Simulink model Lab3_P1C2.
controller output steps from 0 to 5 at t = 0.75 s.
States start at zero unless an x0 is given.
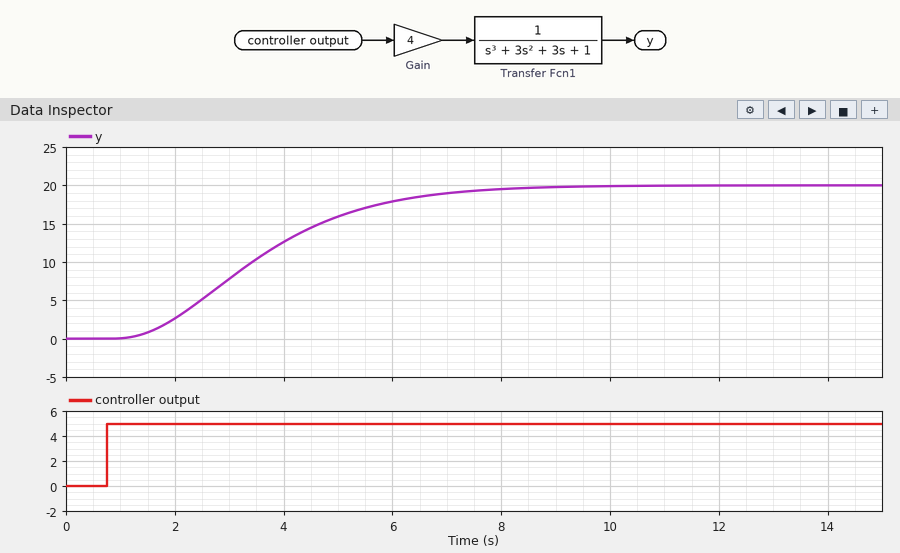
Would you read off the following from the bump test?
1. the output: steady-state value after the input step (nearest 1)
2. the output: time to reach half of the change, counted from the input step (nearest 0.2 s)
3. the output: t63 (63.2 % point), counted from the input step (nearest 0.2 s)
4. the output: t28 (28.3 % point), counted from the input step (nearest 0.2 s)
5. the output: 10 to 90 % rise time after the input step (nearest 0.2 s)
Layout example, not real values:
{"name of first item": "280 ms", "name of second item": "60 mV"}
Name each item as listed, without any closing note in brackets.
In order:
{"the output: steady-state value after the input step": "20", "the output: time to reach half of the change, counted from the input step": "2.6 s", "the output: t63 (63.2 % point), counted from the input step": "3.2 s", "the output: t28 (28.3 % point), counted from the input step": "1.8 s", "the output: 10 to 90 % rise time after the input step": "4.2 s"}
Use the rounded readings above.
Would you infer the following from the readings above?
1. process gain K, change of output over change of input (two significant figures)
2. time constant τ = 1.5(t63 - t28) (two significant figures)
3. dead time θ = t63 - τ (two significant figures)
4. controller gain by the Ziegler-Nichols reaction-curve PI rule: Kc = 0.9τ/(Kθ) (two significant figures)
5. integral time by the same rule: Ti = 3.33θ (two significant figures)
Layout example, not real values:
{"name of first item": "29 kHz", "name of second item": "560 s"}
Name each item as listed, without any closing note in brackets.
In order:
{"process gain K, change of output over change of input": "4.0", "time constant τ = 1.5(t63 - t28)": "2.1 s", "dead time θ = t63 - τ": "1.1 s", "controller gain by the Ziegler-Nichols reaction-curve PI rule: Kc = 0.9τ/(Kθ)": "0.43", "integral time by the same rule: Ti = 3.33θ": "3.7 s"}
